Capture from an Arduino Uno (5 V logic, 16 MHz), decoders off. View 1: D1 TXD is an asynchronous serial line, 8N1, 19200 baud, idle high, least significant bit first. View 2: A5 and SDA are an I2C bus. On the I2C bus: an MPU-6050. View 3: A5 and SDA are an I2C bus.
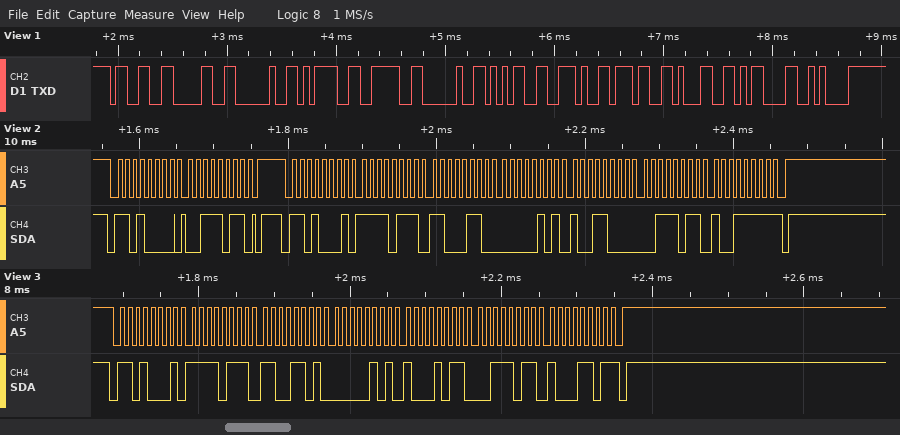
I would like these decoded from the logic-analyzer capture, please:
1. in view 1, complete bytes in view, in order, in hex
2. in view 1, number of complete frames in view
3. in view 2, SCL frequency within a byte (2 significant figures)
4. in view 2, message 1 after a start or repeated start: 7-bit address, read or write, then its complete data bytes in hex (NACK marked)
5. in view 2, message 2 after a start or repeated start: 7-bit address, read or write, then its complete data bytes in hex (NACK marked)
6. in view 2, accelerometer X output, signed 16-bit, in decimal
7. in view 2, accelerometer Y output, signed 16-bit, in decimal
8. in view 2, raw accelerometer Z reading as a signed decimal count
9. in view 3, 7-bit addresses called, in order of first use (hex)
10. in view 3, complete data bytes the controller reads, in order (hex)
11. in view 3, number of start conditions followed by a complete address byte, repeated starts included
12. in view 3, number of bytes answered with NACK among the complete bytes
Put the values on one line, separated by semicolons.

33 30 20 3D 3E 20 35 2E 37 31 0D 0A; 12; 100 kHz; 0x68 write: 3B; 0x68 read: F7 C6 05 98 3B 9F NACK; -2106; 1432; 15263; 0x68; F7 CD 05 8B 3B 8D; 1; 1
